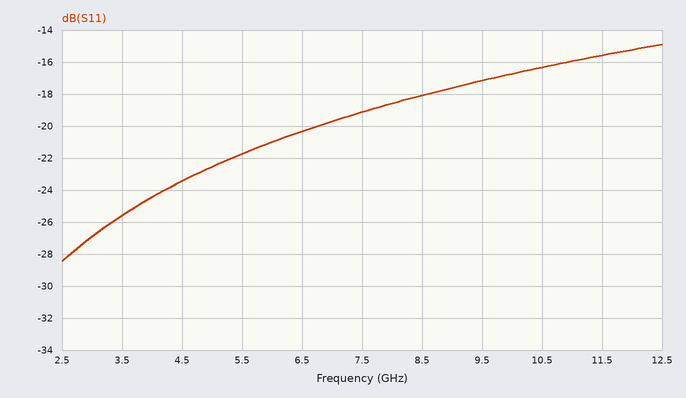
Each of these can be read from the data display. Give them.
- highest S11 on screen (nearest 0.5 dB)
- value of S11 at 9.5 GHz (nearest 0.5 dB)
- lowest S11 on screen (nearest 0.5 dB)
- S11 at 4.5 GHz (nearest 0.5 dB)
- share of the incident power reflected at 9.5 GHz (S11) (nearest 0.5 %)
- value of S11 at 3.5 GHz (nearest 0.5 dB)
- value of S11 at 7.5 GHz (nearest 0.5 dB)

-15.0 dB
-17.0 dB
-28.5 dB
-23.5 dB
2.0 %
-25.5 dB
-19.0 dB
